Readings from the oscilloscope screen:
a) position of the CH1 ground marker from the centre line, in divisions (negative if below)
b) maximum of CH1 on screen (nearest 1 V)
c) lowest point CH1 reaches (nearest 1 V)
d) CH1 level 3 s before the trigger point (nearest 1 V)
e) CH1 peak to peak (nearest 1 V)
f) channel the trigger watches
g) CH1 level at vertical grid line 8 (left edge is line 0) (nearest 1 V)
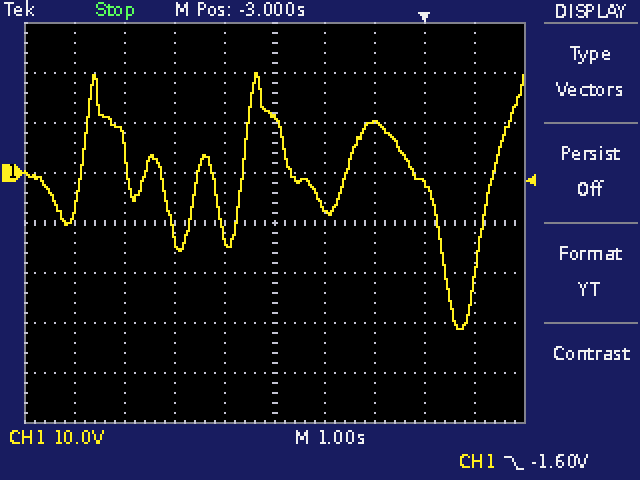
+1.0 div
20 V
-31 V
11 V
51 V
CH1
-2 V
